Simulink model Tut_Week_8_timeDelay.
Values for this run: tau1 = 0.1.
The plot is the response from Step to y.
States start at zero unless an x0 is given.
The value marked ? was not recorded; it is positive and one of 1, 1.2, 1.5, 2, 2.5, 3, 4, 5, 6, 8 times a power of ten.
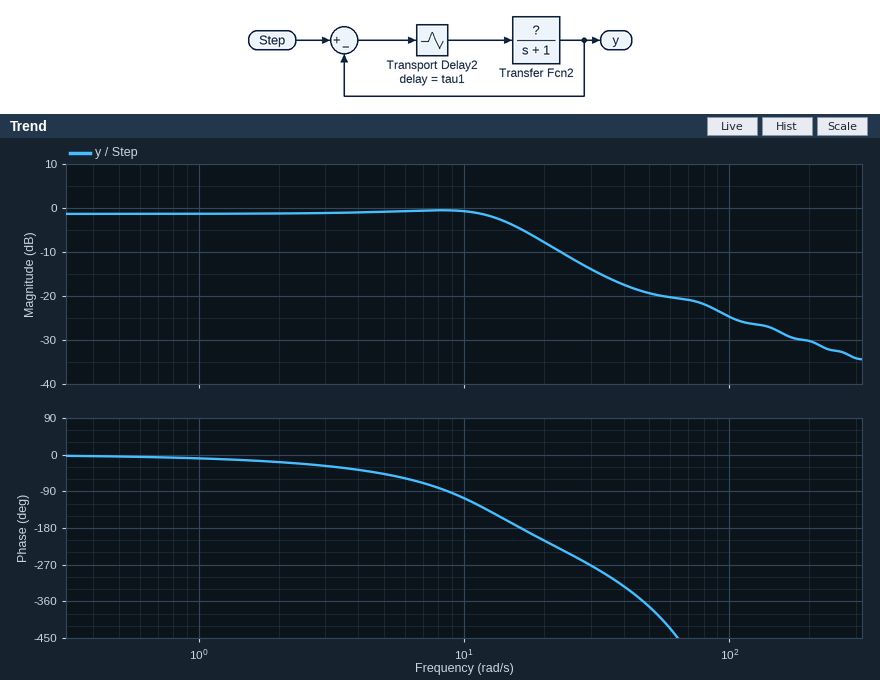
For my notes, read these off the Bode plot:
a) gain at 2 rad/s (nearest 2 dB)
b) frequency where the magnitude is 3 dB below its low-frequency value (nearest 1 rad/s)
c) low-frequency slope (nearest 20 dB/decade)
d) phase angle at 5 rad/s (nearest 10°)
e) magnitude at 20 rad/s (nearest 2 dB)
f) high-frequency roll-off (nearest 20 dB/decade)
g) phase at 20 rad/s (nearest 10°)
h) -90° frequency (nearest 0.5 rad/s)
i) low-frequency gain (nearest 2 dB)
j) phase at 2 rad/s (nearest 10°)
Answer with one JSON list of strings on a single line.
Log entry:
["-2 dB", "16 rad/s", "0 dB/decade", "-50°", "-8 dB", "-20 dB/decade", "-210°", "8.5 rad/s", "-2 dB", "-20°"]
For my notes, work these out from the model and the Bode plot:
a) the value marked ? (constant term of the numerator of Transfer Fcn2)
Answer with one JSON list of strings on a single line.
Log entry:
["6"]
